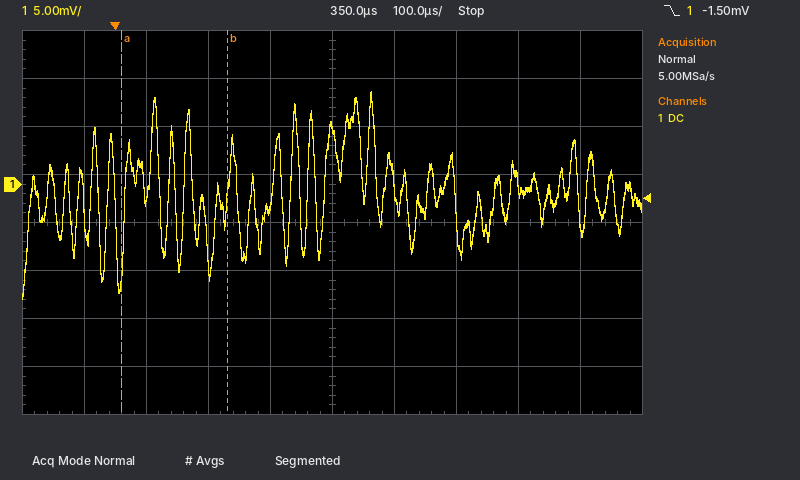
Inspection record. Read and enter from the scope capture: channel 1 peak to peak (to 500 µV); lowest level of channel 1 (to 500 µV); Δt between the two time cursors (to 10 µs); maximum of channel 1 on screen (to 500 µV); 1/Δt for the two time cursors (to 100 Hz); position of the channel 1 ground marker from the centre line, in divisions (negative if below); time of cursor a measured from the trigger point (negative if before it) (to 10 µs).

21.5 mV
-12.0 mV
170 µs
9.5 mV
5.9 kHz
+0.8 div
+10 µs
